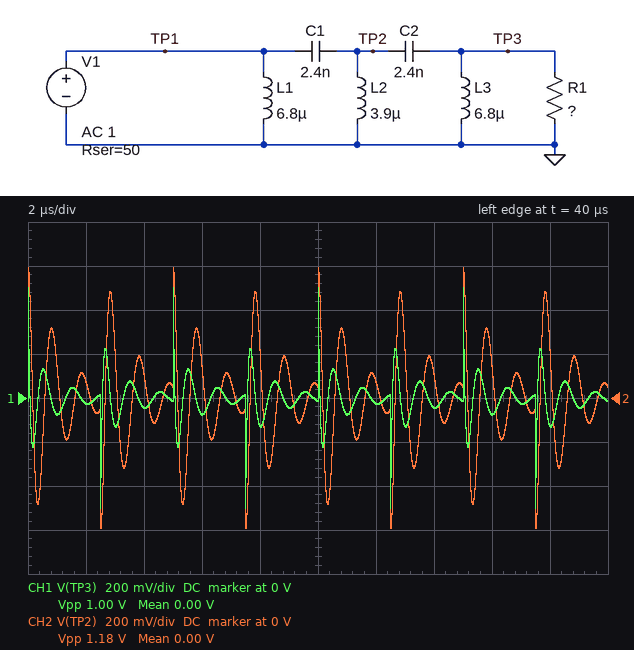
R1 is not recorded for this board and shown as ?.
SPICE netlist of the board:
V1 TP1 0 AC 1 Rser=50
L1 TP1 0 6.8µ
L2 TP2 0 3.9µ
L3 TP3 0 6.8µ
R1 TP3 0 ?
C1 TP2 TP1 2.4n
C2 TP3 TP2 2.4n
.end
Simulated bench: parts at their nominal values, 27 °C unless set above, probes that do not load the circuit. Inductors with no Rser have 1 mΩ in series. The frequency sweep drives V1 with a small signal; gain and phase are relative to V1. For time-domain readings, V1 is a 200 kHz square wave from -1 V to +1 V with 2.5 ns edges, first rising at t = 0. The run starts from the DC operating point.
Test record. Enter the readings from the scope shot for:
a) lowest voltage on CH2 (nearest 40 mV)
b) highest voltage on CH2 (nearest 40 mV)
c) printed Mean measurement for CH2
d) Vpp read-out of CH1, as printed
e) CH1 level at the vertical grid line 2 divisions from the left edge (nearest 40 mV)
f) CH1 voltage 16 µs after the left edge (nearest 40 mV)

-600 mV
600 mV
0.00 V
1.00 V
-40 mV
-80 mV
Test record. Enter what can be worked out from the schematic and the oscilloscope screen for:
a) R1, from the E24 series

18 Ω
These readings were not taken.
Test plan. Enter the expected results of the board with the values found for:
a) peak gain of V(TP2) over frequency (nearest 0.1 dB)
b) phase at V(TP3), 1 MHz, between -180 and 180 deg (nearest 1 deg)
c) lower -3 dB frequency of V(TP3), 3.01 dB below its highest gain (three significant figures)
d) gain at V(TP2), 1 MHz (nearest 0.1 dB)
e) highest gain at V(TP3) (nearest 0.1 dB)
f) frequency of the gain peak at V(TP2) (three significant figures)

-0.5 dB
-125 deg
934 kHz
-0.6 dB
-11.0 dB
1.03 MHz
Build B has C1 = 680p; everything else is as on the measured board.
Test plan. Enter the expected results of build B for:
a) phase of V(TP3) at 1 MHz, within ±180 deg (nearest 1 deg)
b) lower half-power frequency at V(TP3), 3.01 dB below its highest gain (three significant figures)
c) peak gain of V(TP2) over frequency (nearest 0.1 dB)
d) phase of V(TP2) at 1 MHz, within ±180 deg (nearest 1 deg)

-50 deg
1.34 MHz
-5.1 dB
-149 deg
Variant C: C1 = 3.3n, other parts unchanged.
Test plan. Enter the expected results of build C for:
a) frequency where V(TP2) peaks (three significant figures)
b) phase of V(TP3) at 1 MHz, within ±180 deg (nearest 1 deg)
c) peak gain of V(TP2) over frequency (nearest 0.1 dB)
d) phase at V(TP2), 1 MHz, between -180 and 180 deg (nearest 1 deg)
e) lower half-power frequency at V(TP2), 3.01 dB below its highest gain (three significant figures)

898 kHz
-160 deg
-1.0 dB
101 deg
777 kHz
